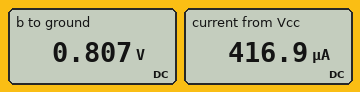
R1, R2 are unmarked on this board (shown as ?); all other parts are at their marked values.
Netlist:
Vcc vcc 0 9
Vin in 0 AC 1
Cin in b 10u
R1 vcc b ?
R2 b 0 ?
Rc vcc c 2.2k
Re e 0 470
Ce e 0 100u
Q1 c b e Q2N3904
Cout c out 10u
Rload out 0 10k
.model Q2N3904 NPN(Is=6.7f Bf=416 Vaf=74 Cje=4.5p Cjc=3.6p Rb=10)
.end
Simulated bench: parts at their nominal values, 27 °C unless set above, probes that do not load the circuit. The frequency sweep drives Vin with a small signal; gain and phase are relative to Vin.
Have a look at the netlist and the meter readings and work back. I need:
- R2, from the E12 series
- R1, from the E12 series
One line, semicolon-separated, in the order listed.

15 kΩ; 150 kΩ
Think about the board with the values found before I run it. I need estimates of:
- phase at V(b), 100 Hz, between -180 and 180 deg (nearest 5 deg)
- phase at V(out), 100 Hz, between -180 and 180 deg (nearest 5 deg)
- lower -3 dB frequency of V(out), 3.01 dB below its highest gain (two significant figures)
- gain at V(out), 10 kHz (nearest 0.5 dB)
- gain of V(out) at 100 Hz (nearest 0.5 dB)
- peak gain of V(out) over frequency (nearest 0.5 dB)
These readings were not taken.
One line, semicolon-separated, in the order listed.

0 deg; -165 deg; 26 Hz; 28.0 dB; 27.5 dB; 28.0 dB
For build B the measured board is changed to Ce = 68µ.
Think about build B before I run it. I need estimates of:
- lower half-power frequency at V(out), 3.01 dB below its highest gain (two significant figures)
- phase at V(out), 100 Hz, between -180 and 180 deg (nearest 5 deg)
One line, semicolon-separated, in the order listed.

37 Hz; -160 deg
